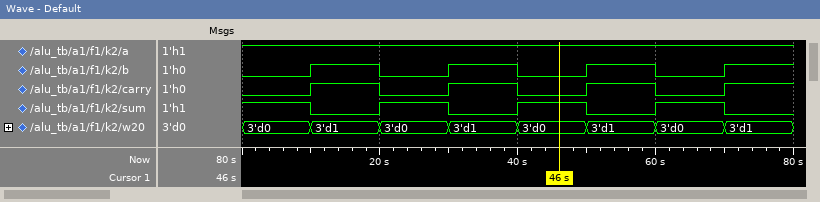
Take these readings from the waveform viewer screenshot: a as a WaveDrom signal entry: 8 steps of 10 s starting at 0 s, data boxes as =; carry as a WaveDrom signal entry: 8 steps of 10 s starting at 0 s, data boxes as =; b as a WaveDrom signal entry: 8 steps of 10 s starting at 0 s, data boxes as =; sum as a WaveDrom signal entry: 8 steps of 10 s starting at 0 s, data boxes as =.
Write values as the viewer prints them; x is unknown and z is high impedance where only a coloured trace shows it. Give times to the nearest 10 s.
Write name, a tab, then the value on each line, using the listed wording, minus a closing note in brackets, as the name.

a as a WaveDrom signal entry: 8 steps of 10 s starting at 0 s, data boxes as =	{name: 'a', wave: '1.......'}
carry as a WaveDrom signal entry: 8 steps of 10 s starting at 0 s, data boxes as =	{name: 'carry', wave: '01010101'}
b as a WaveDrom signal entry: 8 steps of 10 s starting at 0 s, data boxes as =	{name: 'b', wave: '01010101'}
sum as a WaveDrom signal entry: 8 steps of 10 s starting at 0 s, data boxes as =	{name: 'sum', wave: '10101010'}
